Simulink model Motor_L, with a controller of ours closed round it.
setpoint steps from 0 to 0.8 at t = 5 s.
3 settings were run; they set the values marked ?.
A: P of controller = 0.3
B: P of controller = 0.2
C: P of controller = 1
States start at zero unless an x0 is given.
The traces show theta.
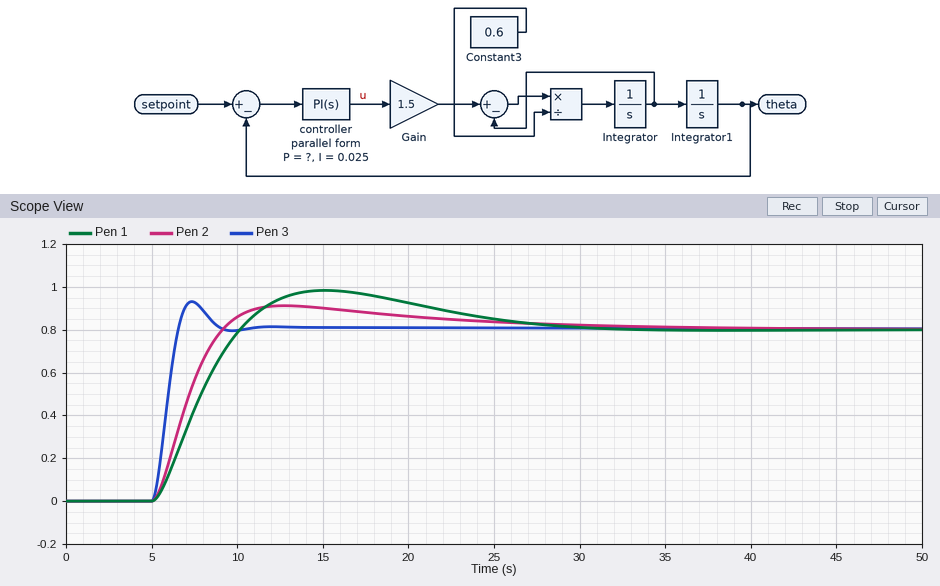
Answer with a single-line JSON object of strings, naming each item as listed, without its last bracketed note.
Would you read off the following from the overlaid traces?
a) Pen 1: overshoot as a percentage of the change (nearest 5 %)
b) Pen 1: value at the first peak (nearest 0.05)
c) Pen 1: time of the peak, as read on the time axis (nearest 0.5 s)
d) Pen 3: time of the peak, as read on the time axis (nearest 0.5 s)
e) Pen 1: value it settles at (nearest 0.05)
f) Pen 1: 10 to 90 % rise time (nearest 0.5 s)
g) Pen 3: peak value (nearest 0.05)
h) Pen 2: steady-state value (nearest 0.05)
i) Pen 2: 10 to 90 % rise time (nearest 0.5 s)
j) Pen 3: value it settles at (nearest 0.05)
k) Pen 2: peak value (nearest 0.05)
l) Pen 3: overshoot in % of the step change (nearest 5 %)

{"Pen 1: overshoot as a percentage of the change": "25 %", "Pen 1: value at the first peak": "1.00", "Pen 1: time of the peak, as read on the time axis": "15.0 s", "Pen 3: time of the peak, as read on the time axis": "7.5 s", "Pen 1: value it settles at": "0.80", "Pen 1: 10 to 90 % rise time": "3.5 s", "Pen 3: peak value": "0.95", "Pen 2: steady-state value": "0.80", "Pen 2: 10 to 90 % rise time": "3.0 s", "Pen 3: value it settles at": "0.80", "Pen 2: peak value": "0.90", "Pen 3: overshoot in % of the step change": "15 %"}
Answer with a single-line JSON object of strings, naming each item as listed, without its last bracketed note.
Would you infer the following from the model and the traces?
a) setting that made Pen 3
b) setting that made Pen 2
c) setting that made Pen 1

{"setting that made Pen 3": "C", "setting that made Pen 2": "A", "setting that made Pen 1": "B"}
